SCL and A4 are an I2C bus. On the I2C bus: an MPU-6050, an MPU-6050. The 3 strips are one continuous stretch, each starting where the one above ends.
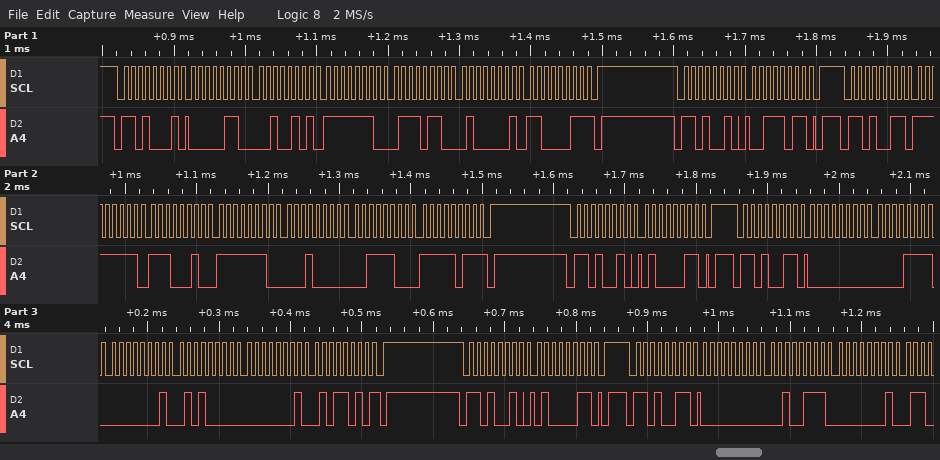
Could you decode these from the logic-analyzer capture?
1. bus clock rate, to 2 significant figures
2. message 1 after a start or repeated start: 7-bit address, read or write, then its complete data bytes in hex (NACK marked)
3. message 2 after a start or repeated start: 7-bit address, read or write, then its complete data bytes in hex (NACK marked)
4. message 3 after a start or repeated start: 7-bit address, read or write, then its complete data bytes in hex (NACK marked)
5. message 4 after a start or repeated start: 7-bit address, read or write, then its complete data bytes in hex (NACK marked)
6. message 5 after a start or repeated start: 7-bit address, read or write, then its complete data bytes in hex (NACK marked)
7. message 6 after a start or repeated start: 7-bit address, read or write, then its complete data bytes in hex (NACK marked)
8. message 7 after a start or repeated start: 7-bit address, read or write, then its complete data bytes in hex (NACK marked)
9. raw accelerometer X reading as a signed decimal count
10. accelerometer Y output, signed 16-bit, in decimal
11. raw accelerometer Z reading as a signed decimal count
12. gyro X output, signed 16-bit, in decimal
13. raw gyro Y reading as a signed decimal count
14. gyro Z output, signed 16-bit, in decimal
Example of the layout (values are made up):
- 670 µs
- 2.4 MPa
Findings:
- 100 kHz
- 0x68 read: 06 25 FE 76 41 C3 NACK
- 0x69 write: 3B
- 0x69 read: FF E2 FE 10 3C FB NACK
- 0x69 write: 43
- 0x69 read: 00 0F 01 50 01 5A NACK
- 0x69 write: 43
- 0x69 read: 00 27 01
- -30
- -496
- 15611
- 15
- 336
- 346
